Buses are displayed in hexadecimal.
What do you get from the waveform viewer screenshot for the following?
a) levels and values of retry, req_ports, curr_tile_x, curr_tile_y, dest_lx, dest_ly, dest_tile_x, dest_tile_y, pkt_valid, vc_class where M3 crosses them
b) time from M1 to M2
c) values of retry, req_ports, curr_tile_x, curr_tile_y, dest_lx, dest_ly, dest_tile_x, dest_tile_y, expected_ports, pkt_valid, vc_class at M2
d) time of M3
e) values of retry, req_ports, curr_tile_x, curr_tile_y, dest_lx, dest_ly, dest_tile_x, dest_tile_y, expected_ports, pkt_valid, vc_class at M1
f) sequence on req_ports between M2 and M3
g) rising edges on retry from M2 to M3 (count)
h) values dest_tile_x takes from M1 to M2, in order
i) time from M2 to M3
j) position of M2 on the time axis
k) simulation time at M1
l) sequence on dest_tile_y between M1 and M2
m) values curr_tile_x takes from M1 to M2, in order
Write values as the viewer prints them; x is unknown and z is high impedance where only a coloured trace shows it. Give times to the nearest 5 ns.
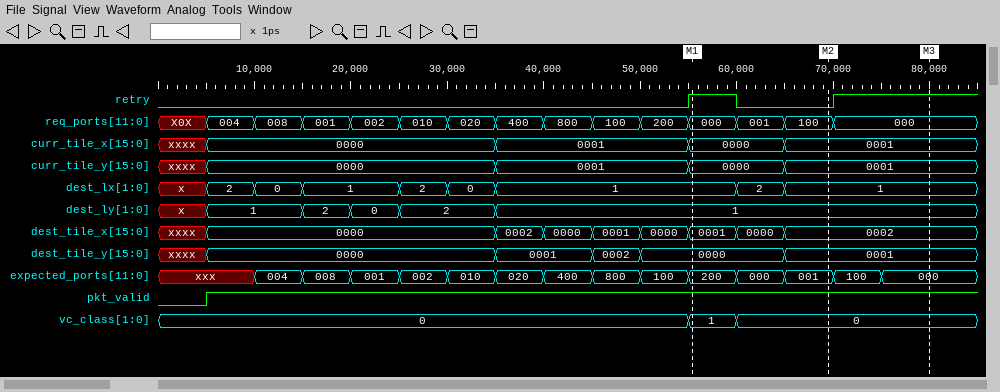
retry=1, req_ports=000, curr_tile_x=0001, curr_tile_y=0001, dest_lx=1, dest_ly=1, dest_tile_x=0002, dest_tile_y=0001, pkt_valid=1, vc_class=0
15 ns
retry=0, req_ports=100, curr_tile_x=0001, curr_tile_y=0001, dest_lx=1, dest_ly=1, dest_tile_x=0002, dest_tile_y=0001, expected_ports=001, pkt_valid=1, vc_class=0
80 ns
retry=1, req_ports=000, curr_tile_x=0000, curr_tile_y=0000, dest_lx=1, dest_ly=1, dest_tile_x=0001, dest_tile_y=0000, expected_ports=200, pkt_valid=1, vc_class=1
100, 000
1
0001, 0000, 0002
10 ns
70 ns
55 ns
0000, 0001
0000, 0001
